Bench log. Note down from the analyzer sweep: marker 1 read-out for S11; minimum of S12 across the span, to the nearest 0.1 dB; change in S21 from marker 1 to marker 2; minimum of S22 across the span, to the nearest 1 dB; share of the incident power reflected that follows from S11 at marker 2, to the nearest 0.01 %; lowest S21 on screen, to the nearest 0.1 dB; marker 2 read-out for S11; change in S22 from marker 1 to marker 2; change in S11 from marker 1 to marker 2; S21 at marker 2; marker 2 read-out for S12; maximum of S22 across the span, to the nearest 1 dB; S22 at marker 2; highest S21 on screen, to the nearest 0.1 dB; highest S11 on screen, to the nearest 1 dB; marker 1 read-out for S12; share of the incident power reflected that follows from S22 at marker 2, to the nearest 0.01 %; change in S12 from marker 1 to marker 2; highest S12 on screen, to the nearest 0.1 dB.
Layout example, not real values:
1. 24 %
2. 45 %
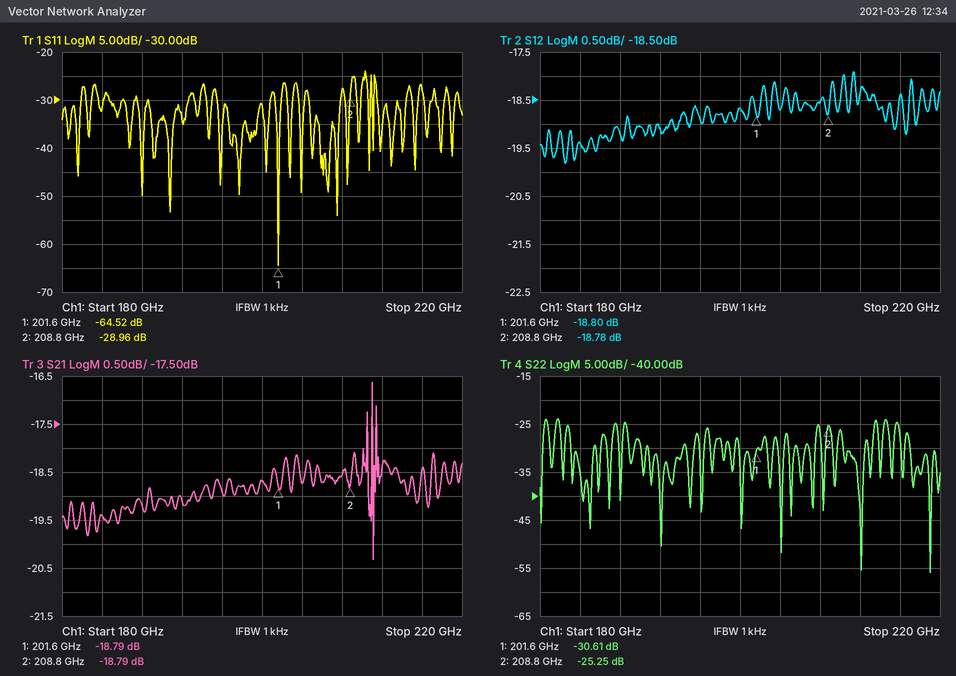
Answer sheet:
1. -64.52 dB
2. -19.8 dB
3. 0.00 dB
4. -56 dB
5. 0.13 %
6. -20.3 dB
7. -28.96 dB
8. 5.36 dB
9. 35.56 dB
10. -18.79 dB
11. -18.78 dB
12. -24 dB
13. -25.25 dB
14. -16.6 dB
15. -24 dB
16. -18.80 dB
17. 0.30 %
18. 0.02 dB
19. -17.9 dB
